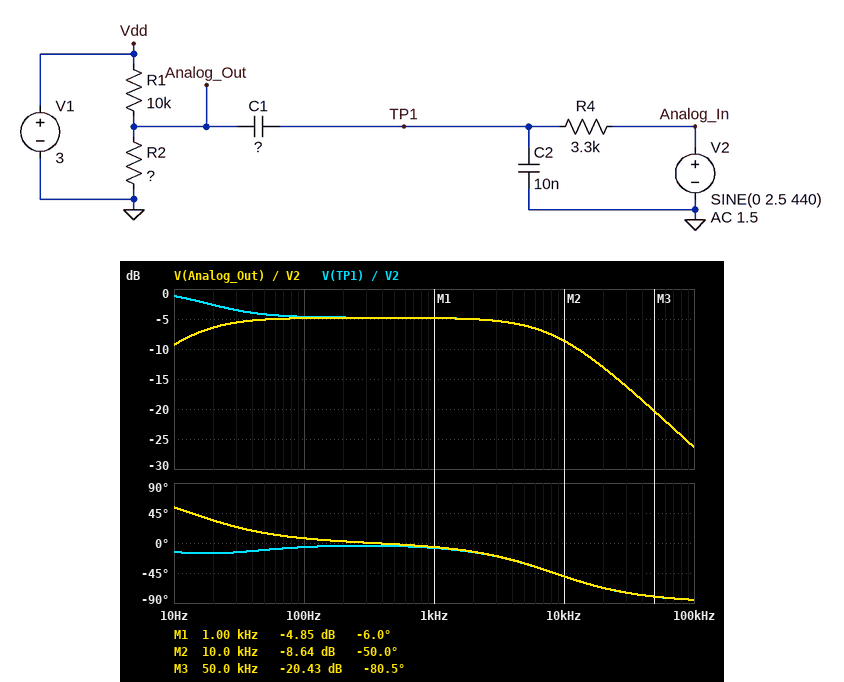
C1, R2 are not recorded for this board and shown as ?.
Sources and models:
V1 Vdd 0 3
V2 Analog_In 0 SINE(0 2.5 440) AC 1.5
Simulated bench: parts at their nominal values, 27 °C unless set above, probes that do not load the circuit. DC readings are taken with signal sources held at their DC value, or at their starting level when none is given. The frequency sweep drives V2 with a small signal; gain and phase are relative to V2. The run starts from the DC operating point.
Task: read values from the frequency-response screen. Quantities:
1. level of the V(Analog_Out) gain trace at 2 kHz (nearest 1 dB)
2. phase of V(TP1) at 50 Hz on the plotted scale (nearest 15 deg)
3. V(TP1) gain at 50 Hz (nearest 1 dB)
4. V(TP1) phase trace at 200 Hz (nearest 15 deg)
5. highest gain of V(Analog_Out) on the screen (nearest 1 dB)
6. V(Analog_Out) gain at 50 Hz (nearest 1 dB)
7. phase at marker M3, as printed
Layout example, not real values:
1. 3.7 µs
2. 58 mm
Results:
1. -5 dB
2. -15 deg
3. -4 dB
4. 0 deg
5. -5 dB
6. -5 dB
7. -80.5 deg
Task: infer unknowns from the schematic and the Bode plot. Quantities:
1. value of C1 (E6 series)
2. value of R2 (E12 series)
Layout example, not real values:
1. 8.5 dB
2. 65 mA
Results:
1. 1.5 µF
2. 8.2 kΩ
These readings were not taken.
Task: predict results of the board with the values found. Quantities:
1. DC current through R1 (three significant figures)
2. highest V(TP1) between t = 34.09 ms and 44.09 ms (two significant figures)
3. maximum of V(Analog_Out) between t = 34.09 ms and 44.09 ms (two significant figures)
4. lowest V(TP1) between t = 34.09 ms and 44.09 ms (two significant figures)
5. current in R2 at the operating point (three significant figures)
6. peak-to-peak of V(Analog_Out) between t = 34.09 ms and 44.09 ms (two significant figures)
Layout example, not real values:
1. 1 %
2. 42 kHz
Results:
1. 165 µA
2. 1.4 V
3. 2.8 V
4. -1.4 V
5. 165 µA
6. 2.9 V
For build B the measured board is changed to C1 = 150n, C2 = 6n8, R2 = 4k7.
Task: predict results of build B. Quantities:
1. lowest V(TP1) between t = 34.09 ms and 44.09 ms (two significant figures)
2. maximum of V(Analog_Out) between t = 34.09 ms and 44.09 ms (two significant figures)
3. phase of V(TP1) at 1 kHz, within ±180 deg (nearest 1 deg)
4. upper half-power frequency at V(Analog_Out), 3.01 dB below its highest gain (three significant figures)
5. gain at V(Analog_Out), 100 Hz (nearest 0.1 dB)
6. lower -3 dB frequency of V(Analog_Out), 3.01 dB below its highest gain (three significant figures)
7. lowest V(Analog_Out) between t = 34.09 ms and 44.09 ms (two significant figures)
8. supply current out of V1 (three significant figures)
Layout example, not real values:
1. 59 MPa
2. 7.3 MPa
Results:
1. -1.4 V
2. 2.1 V
3. -13 deg
4. 14.9 kHz
5. -11.8 dB
6. 158 Hz
7. -180 mV
8. 204 µA
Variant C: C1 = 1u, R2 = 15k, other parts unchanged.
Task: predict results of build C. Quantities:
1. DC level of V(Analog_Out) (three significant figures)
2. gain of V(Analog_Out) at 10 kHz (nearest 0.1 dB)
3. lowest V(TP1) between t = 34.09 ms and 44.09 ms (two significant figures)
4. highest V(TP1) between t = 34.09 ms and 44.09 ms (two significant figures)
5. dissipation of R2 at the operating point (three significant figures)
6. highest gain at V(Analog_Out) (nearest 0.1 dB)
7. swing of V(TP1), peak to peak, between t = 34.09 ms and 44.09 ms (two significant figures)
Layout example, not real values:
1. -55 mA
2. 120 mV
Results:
1. 1.80 V
2. -8.3 dB
3. -1.6 V
4. 1.6 V
5. 216 µW
6. -3.8 dB
7. 3.2 V
